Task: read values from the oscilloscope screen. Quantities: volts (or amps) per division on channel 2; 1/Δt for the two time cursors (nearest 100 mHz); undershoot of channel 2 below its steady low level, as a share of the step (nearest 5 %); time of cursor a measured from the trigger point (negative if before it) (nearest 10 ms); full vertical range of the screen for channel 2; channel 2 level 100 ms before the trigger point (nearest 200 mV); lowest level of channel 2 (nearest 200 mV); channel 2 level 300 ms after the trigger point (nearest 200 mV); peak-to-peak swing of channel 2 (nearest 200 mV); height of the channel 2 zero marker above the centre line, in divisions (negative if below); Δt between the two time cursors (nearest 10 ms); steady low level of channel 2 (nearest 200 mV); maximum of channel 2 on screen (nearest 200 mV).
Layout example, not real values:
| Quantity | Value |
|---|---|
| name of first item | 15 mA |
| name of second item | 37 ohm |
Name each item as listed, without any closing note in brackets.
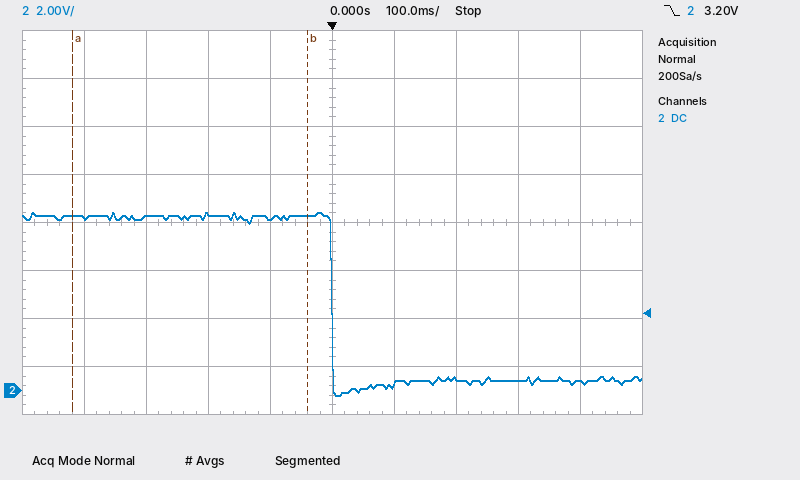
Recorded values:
| Quantity | Value |
|---|---|
| volts (or amps) per division on channel 2 | 2 V |
| 1/Δt for the two time cursors | 2.6 Hz |
| undershoot of channel 2 below its steady low level, as a share of the step | 10 % |
| time of cursor a measured from the trigger point (negative if before it) | -420 ms |
| full vertical range of the screen for channel 2 | 16 V |
| channel 2 level 100 ms before the trigger point | 7.2 V |
| lowest level of channel 2 | -200 mV |
| channel 2 level 300 ms after the trigger point | 400 mV |
| peak-to-peak swing of channel 2 | 7.6 V |
| height of the channel 2 zero marker above the centre line, in divisions | -3.5 div |
| Δt between the two time cursors | 380 ms |
| steady low level of channel 2 | 400 mV |
| maximum of channel 2 on screen | 7.4 V |
